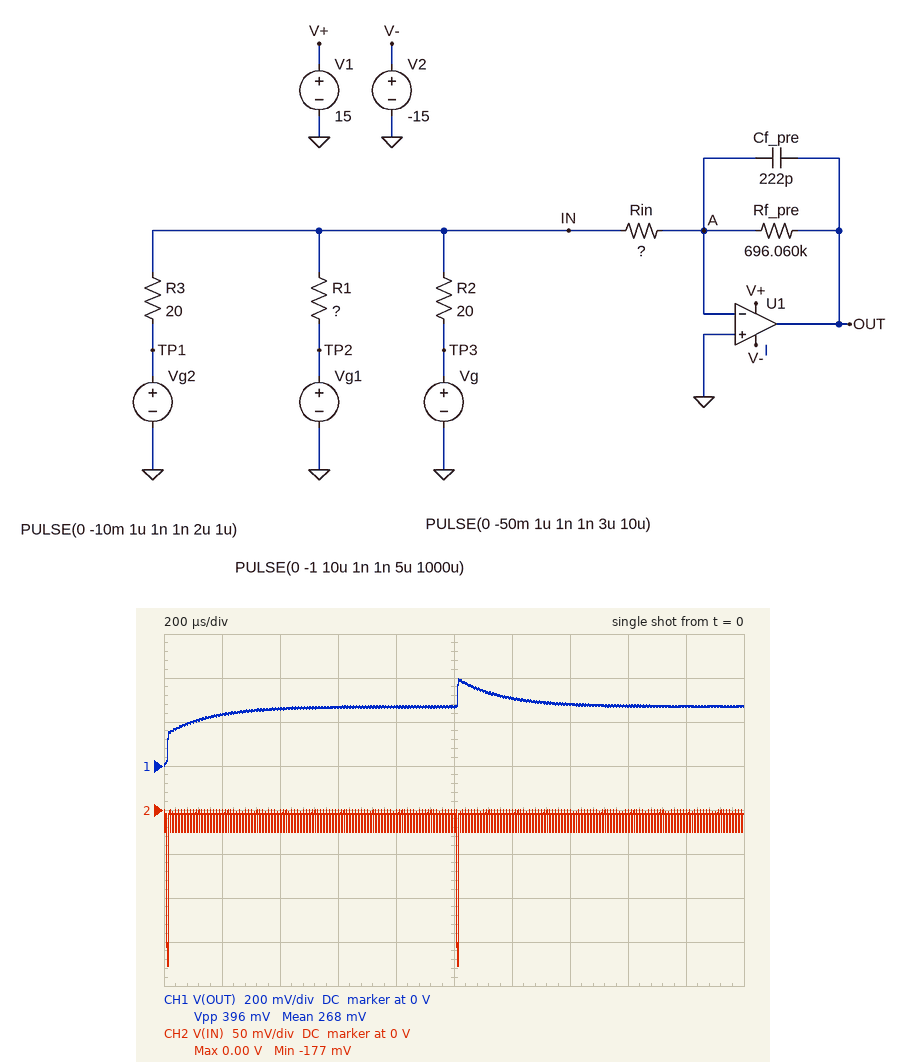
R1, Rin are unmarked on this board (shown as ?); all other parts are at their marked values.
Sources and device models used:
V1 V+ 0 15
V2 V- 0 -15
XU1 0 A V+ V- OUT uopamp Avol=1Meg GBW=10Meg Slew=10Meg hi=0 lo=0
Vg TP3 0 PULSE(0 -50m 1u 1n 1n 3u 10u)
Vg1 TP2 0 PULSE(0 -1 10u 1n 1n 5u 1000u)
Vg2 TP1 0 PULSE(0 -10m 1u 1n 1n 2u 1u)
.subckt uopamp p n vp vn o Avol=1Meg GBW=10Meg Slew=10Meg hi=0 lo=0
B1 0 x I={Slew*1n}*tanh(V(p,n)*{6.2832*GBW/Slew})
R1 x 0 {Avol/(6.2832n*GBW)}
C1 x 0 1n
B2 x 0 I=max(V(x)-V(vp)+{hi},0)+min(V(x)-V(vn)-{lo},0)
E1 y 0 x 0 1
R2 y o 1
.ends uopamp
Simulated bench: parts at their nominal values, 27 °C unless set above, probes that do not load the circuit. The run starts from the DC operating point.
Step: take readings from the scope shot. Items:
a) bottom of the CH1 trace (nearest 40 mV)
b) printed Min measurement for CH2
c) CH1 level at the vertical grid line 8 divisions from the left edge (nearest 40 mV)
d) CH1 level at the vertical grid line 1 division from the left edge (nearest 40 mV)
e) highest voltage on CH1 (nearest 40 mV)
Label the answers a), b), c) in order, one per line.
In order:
a) 0 V
b) -177 mV
c) 280 mV
d) 240 mV
e) 400 mV
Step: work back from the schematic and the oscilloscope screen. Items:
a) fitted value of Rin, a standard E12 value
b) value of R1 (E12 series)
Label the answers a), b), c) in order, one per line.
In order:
a) 27 kΩ
b) 56 Ω
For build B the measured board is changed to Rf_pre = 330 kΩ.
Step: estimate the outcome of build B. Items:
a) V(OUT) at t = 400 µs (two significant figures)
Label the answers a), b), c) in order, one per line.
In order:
a) 130 mV
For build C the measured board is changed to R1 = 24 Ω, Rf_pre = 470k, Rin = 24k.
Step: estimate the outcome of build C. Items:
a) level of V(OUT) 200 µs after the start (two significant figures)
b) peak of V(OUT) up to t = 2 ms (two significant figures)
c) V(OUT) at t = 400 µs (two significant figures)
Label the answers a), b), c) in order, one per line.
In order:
a) 190 mV
b) 440 mV
c) 170 mV
